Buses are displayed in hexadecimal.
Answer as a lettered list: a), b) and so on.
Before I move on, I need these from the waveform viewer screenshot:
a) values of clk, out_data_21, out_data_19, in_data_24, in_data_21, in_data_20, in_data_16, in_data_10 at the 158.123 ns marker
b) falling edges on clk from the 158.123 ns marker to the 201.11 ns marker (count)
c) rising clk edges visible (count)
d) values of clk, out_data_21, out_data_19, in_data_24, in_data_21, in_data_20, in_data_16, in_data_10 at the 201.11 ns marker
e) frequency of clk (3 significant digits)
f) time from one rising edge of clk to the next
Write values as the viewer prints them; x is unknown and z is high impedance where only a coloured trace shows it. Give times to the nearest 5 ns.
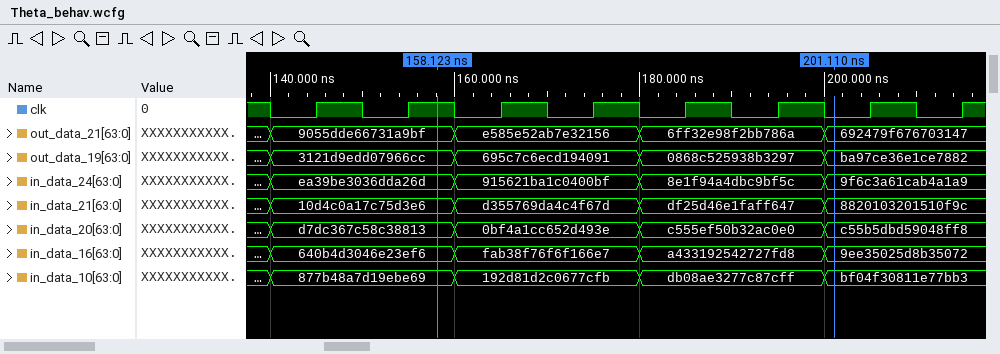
a) clk=1, out_data_21=9055dde66731a9bf, out_data_19=3121d9edd07966cc, in_data_24=ea39be3036dda26d, in_data_21=10d4c0a17c75d3e6, in_data_20=d7dc367c58c38813, in_data_16=640b4d3046e23ef6, in_data_10=877b48a7d19ebe69
b) 5
c) 8
d) clk=0, out_data_21=692479f676703147, out_data_19=ba97ce36e1ce7882, in_data_24=9f6c3a61cab4a1a9, in_data_21=8820103201510f9c, in_data_20=c55b5dbd59048ff8, in_data_16=9ee35025d8b35072, in_data_10=bf04f30811e77bb3
e) 100 MHz
f) 10 ns
